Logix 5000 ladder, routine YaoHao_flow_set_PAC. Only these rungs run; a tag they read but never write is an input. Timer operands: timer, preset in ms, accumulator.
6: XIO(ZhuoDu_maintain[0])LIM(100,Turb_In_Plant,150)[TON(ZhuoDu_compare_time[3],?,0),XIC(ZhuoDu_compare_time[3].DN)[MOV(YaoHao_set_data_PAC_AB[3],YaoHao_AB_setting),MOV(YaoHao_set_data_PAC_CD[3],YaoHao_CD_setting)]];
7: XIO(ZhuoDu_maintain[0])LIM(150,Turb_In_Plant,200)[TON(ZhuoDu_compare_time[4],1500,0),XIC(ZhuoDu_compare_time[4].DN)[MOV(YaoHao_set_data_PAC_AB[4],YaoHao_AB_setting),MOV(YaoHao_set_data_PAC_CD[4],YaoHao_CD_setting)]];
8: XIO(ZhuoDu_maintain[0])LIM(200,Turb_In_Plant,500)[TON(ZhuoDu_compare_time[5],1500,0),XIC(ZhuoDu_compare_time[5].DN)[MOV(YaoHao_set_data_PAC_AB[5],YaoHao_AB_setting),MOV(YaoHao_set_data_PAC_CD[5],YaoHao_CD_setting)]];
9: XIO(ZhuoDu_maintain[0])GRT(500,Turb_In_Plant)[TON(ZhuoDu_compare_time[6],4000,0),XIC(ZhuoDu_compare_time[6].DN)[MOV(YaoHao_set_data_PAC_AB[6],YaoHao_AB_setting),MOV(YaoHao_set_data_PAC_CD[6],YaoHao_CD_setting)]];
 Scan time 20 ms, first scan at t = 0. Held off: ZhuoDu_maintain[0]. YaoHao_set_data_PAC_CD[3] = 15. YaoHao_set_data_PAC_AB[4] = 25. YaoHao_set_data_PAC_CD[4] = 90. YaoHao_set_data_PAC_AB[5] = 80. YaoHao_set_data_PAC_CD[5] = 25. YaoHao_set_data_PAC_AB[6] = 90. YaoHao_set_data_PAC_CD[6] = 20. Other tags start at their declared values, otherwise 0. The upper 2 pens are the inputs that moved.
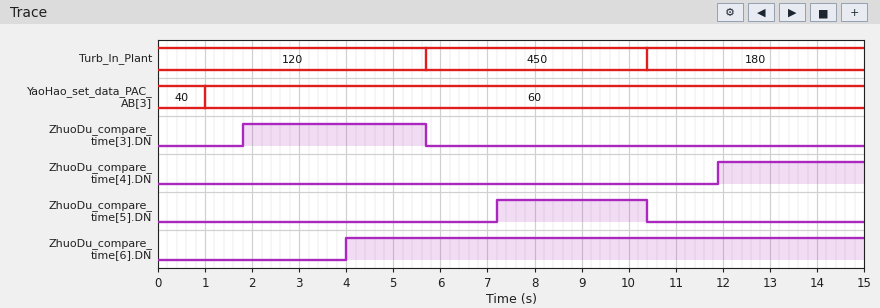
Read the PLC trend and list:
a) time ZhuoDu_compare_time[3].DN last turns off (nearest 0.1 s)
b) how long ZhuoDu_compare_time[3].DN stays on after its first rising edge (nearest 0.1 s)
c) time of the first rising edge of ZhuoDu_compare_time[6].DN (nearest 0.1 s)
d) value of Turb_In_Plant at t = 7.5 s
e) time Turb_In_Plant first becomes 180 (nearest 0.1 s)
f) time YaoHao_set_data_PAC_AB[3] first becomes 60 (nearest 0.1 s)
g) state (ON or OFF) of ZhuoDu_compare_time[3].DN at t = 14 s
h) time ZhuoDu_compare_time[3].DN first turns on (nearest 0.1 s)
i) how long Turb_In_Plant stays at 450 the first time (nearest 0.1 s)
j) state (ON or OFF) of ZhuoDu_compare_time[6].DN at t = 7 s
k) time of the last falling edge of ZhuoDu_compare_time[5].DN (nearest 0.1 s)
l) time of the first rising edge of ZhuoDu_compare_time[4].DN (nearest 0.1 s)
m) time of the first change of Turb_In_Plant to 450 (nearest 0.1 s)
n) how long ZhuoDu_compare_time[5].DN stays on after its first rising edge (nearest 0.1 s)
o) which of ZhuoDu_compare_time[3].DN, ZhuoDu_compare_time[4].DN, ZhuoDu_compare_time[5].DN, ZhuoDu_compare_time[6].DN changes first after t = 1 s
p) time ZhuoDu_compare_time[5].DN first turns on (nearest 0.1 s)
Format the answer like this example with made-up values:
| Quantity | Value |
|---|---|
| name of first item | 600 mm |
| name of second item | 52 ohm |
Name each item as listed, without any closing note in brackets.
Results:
| Quantity | Value |
|---|---|
| time ZhuoDu_compare_time[3].DN last turns off | 5.7 s |
| how long ZhuoDu_compare_time[3].DN stays on after its first rising edge | 3.9 s |
| time of the first rising edge of ZhuoDu_compare_time[6].DN | 4.0 s |
| value of Turb_In_Plant at t = 7.5 s | 450 |
| time Turb_In_Plant first becomes 180 | 10.4 s |
| time YaoHao_set_data_PAC_AB[3] first becomes 60 | 1.0 s |
| state (ON or OFF) of ZhuoDu_compare_time[3].DN at t = 14 s | OFF |
| time ZhuoDu_compare_time[3].DN first turns on | 1.8 s |
| how long Turb_In_Plant stays at 450 the first time | 4.7 s |
| state (ON or OFF) of ZhuoDu_compare_time[6].DN at t = 7 s | ON |
| time of the last falling edge of ZhuoDu_compare_time[5].DN | 10.4 s |
| time of the first rising edge of ZhuoDu_compare_time[4].DN | 11.9 s |
| time of the first change of Turb_In_Plant to 450 | 5.7 s |
| how long ZhuoDu_compare_time[5].DN stays on after its first rising edge | 3.2 s |
| which of ZhuoDu_compare_time[3].DN, ZhuoDu_compare_time[4].DN, ZhuoDu_compare_time[5].DN, ZhuoDu_compare_time[6].DN changes first after t = 1 s | ZhuoDu_compare_time[3].DN |
| time ZhuoDu_compare_time[5].DN first turns on | 7.2 s |
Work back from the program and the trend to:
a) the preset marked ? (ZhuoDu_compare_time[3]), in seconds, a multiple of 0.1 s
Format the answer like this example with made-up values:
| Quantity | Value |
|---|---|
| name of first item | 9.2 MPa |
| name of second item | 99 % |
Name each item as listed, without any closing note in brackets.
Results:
| Quantity | Value |
|---|---|
| the preset marked ? (ZhuoDu_compare_time[3]), in seconds, a multiple of 0.1 s | 1.8 s |
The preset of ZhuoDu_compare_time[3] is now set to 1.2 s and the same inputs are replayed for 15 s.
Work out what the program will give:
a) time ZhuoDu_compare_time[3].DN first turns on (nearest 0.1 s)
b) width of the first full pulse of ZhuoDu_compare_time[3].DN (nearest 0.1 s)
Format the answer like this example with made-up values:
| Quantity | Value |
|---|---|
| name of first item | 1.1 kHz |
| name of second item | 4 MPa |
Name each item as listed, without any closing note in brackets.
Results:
| Quantity | Value |
|---|---|
| time ZhuoDu_compare_time[3].DN first turns on | 1.2 s |
| width of the first full pulse of ZhuoDu_compare_time[3].DN | 4.5 s |
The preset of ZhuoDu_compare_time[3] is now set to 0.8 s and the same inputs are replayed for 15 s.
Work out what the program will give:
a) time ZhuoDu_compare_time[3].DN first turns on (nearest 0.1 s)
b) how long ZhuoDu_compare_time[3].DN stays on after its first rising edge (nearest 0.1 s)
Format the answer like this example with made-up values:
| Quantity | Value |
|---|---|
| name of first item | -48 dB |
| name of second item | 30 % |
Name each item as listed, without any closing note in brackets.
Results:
| Quantity | Value |
|---|---|
| time ZhuoDu_compare_time[3].DN first turns on | 0.8 s |
| how long ZhuoDu_compare_time[3].DN stays on after its first rising edge | 4.9 s |
